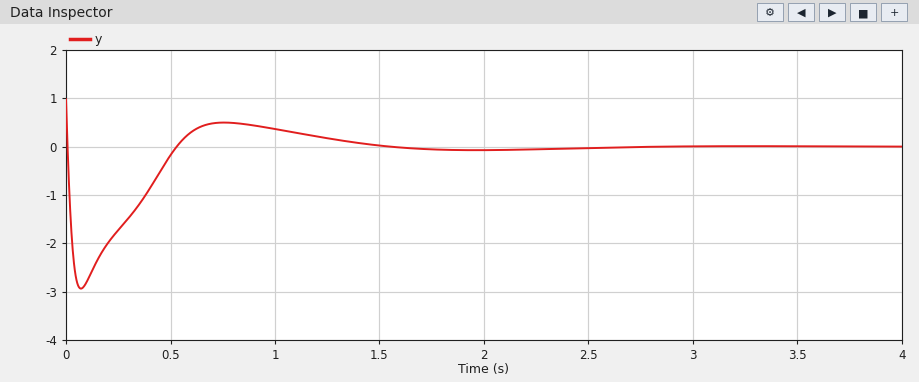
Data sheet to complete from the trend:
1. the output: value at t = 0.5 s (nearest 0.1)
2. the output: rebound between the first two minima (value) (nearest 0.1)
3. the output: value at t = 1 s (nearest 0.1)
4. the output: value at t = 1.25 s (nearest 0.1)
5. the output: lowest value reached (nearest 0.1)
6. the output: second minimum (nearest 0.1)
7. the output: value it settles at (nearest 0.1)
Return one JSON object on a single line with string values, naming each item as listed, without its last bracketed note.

{"the output: value at t = 0.5 s": "-0.2", "the output: rebound between the first two minima (value)": "0.5", "the output: value at t = 1 s": "0.4", "the output: value at t = 1.25 s": "0.2", "the output: lowest value reached": "-2.9", "the output: second minimum": "-0.1", "the output: value it settles at": "0.0"}
